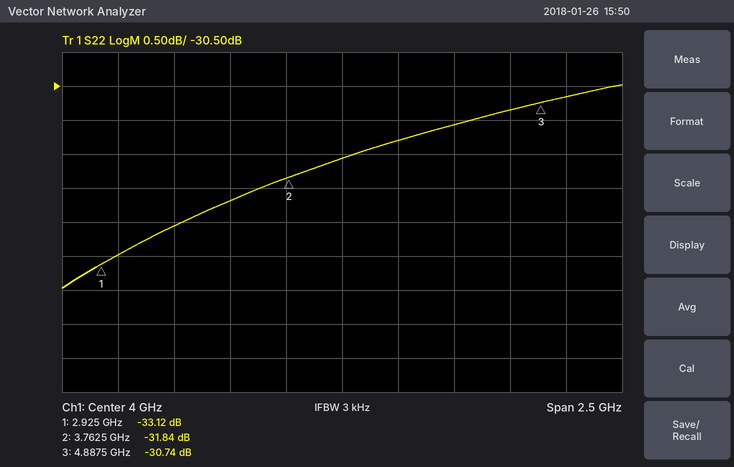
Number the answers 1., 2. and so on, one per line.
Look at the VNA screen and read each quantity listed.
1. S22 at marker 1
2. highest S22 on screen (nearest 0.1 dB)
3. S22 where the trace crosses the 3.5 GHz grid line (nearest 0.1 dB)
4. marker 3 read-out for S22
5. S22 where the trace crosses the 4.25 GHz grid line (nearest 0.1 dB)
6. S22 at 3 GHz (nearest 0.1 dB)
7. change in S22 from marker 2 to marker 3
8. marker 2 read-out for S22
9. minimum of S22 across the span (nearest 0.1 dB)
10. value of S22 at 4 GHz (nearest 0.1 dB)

1. -33.12 dB
2. -30.5 dB
3. -32.2 dB
4. -30.74 dB
5. -31.3 dB
6. -33.0 dB
7. 1.10 dB
8. -31.84 dB
9. -33.5 dB
10. -31.6 dB
